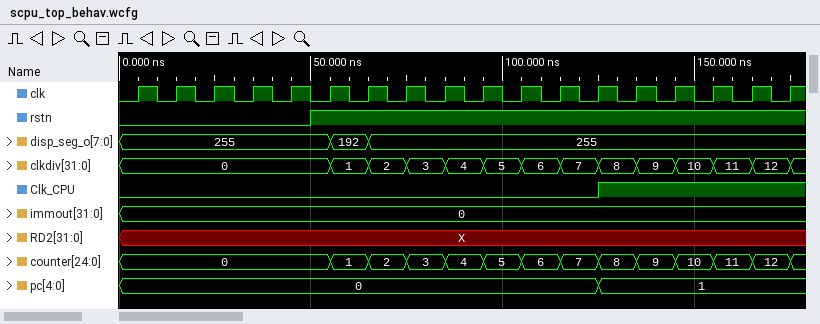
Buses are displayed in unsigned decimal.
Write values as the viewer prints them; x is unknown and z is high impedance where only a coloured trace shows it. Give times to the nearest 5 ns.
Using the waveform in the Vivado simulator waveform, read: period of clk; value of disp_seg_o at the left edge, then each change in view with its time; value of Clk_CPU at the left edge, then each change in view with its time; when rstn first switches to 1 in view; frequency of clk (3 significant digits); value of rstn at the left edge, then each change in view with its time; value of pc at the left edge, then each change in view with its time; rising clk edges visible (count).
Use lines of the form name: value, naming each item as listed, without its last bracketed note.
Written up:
period of clk: 10 ns
value of disp_seg_o at the left edge, then each change in view with its time: 255, 192 at 55 ns, 255 at 65 ns
value of Clk_CPU at the left edge, then each change in view with its time: 0, 1 at 125 ns
when rstn first switches to 1 in view: 50 ns
frequency of clk: 100 MHz
value of rstn at the left edge, then each change in view with its time: 0, 1 at 50 ns
value of pc at the left edge, then each change in view with its time: 0, 1 at 125 ns
rising clk edges visible: 18
